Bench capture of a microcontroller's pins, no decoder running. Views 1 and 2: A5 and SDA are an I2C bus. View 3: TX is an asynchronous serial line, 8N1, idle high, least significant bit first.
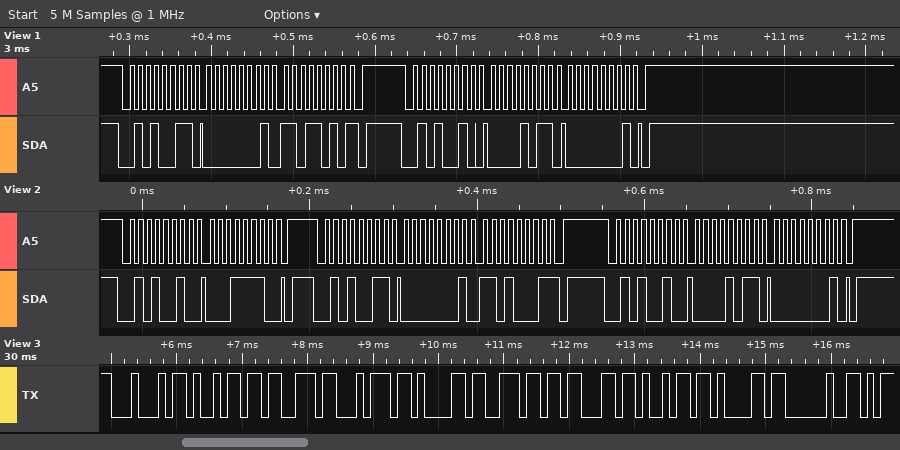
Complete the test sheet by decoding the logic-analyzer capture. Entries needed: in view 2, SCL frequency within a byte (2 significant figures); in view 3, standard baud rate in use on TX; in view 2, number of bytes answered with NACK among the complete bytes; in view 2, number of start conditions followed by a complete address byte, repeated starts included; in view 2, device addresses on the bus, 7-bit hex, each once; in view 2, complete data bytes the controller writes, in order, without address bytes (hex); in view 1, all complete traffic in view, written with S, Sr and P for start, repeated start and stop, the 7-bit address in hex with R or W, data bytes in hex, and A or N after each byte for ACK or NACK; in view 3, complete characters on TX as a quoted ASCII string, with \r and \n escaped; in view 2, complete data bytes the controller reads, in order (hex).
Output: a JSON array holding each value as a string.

["100 kHz", "9600 baud", "1", "3", "0x29", "1E 0B 01", "S 29R A 01 A DA N P S 29W A 0B A 01 A P", "\"Distancia \"", "01 D1"]
